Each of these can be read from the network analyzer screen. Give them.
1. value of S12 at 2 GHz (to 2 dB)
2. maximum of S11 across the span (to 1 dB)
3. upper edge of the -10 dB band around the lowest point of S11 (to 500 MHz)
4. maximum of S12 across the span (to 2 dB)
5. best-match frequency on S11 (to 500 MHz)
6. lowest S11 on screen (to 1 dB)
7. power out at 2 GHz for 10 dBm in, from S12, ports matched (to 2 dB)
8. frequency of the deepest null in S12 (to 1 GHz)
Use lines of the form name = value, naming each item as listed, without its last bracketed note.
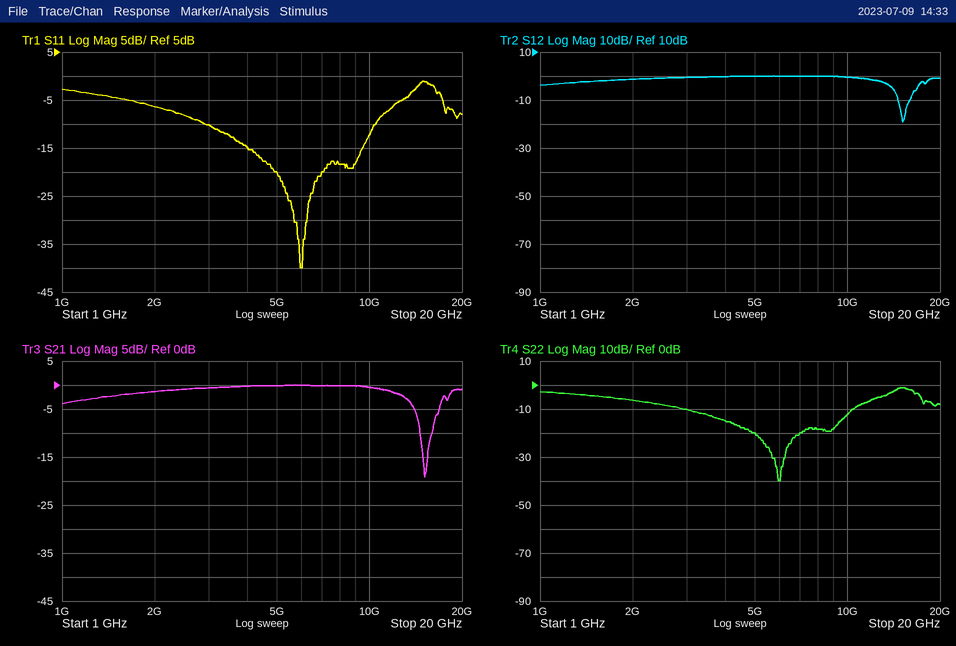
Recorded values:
value of S12 at 2 GHz = -2 dB
maximum of S11 across the span = -1 dB
upper edge of the -10 dB band around the lowest point of S11 = 10.5 GHz
maximum of S12 across the span = 0 dB
best-match frequency on S11 = 6.0 GHz
lowest S11 on screen = -40 dB
power out at 2 GHz for 10 dBm in, from S12, ports matched = 8 dBm
frequency of the deepest null in S12 = 15 GHz
